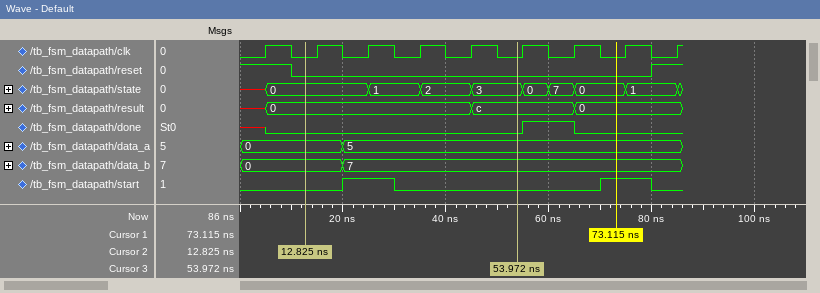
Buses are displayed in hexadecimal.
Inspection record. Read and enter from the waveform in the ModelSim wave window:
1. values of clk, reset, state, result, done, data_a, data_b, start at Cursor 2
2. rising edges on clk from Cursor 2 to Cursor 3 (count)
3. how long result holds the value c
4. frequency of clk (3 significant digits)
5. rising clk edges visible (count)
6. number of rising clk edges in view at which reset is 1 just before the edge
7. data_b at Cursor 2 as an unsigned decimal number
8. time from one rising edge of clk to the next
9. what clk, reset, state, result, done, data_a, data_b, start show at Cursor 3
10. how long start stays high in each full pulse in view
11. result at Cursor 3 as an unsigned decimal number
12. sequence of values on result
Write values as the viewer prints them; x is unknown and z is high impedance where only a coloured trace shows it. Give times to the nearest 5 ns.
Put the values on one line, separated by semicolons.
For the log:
clk=0, reset=0, state=0, result=0, done=0, data_a=0, data_b=0, start=0; 4; 20 ns; 100 MHz; 9; 2; 0; 10 ns; clk=0, reset=0, state=3, result=c, done=0, data_a=5, data_b=7, start=0; 10 ns, 10 ns; 12; x, 0, c, 0
